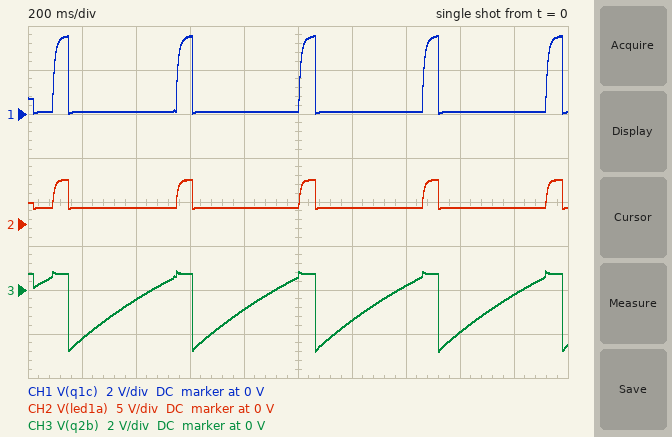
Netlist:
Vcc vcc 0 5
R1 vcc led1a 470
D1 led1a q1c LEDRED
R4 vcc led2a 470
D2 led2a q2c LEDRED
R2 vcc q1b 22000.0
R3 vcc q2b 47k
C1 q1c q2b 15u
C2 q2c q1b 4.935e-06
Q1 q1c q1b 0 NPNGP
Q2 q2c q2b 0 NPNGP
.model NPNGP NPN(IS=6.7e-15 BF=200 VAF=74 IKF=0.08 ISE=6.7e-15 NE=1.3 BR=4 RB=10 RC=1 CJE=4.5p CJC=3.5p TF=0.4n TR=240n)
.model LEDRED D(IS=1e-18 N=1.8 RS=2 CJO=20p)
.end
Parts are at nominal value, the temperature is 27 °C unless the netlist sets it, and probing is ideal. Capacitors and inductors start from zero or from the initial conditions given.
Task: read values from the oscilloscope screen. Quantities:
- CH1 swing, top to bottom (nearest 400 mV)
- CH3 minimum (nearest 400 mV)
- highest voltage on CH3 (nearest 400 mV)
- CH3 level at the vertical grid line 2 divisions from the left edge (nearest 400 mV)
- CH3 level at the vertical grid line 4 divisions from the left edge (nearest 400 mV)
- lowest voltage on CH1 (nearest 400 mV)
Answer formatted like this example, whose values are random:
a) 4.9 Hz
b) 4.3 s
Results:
a) 3.6 V
b) -2.8 V
c) 800 mV
d) -400 mV
e) -800 mV
f) 0 V
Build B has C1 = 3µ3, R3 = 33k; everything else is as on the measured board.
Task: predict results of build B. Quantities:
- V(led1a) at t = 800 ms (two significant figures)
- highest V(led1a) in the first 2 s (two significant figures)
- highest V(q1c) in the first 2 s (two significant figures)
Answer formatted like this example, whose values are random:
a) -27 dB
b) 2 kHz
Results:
a) 5.0 V
b) 5.0 V
c) 3.7 V
